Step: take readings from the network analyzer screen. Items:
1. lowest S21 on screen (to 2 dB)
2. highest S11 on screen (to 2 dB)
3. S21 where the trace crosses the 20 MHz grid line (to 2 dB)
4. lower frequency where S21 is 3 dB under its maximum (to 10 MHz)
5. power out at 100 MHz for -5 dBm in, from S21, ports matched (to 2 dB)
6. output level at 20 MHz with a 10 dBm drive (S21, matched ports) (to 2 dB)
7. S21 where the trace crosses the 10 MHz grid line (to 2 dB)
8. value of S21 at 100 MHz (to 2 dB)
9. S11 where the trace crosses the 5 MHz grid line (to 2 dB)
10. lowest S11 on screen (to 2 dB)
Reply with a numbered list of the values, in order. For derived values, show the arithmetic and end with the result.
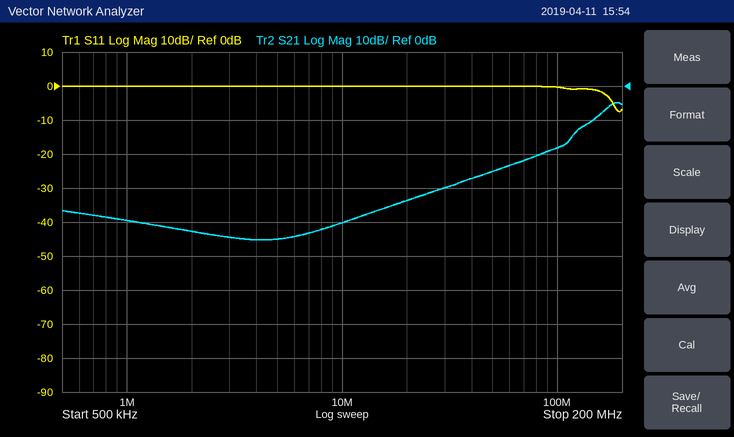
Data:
1. -46 dB
2. 0 dB
3. -34 dB
4. 160 MHz
5. -5 dBm + (-18 dB) = -24 dBm
6. 10 dBm + (-34 dB) = -24 dBm
7. -40 dB
8. -18 dB
9. 0 dB
10. -8 dB
